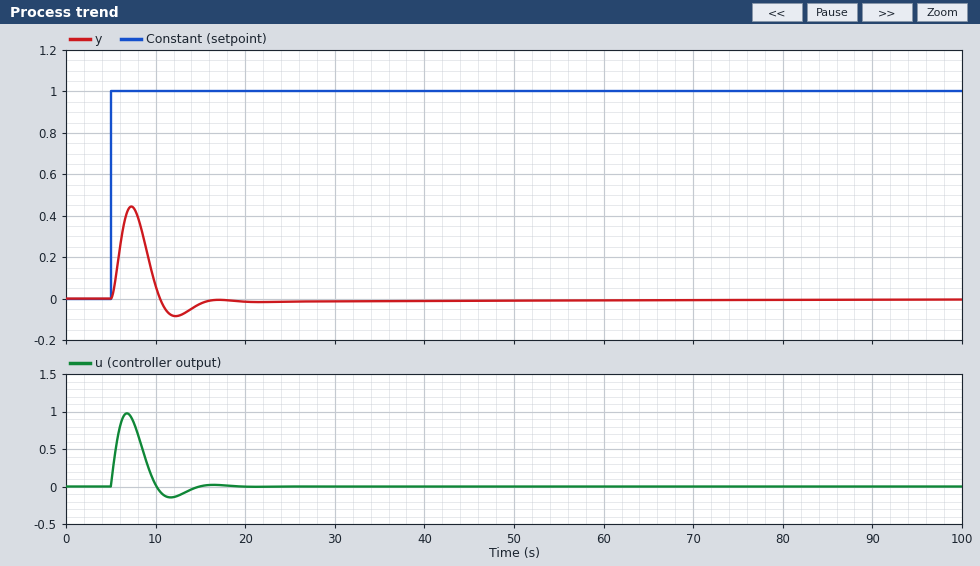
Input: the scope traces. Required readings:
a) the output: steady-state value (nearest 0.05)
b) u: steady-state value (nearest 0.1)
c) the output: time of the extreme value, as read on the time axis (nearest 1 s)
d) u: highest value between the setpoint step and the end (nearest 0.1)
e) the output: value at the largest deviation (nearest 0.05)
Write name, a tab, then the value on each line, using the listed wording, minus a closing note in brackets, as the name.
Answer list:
the output: steady-state value	0.00
u: steady-state value	0.0
the output: time of the extreme value, as read on the time axis	7 s
u: highest value between the setpoint step and the end	1.0
the output: value at the largest deviation	0.45
